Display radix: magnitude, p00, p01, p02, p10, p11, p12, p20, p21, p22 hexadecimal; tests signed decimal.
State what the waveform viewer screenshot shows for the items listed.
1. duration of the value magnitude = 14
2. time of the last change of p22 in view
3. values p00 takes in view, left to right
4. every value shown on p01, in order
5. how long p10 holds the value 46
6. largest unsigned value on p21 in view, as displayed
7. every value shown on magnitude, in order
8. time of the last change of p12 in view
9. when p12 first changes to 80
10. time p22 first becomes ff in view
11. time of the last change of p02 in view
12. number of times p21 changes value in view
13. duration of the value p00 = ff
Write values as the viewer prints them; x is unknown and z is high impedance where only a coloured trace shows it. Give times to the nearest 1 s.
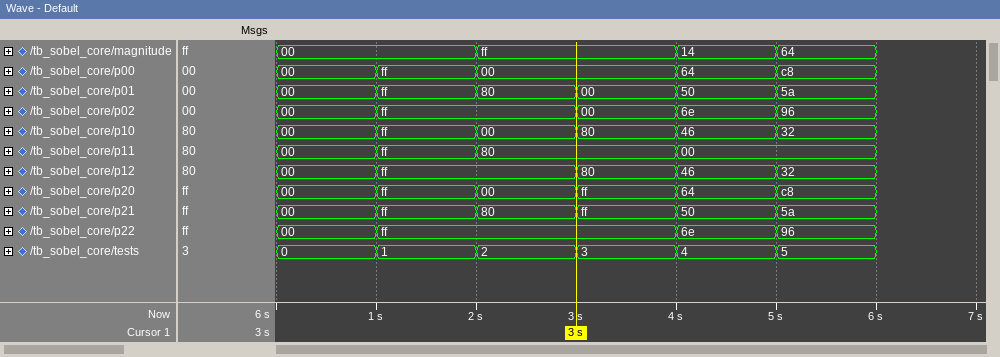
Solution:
1 s
5 s
00, ff, 00, 64, c8
00, ff, 80, 00, 50, 5a
1 s
ff
00, ff, 14, 64
5 s
3 s
1 s
5 s
5
1 s
